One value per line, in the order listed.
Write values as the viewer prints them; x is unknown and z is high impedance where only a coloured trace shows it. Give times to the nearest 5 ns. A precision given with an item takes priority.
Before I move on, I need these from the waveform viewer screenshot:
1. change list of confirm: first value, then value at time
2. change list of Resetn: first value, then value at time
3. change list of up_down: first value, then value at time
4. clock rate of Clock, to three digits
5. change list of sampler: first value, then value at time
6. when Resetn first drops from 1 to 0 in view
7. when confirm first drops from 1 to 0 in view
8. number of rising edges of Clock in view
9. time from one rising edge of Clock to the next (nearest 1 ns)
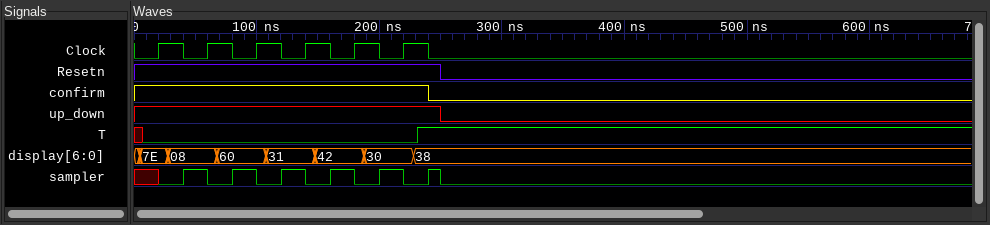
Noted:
1, 0 at 240 ns
1, 0 at 250 ns
1, 0 at 250 ns
25.0 MHz
x, 0 at 20 ns, 1 at 40 ns, 0 at 60 ns, 1 at 80 ns, 0 at 100 ns, 1 at 120 ns, 0 at 140 ns, 1 at 160 ns, 0 at 180 ns, 1 at 200 ns, 0 at 220 ns, 1 at 240 ns, 0 at 250 ns
250 ns
240 ns
6
40 ns
